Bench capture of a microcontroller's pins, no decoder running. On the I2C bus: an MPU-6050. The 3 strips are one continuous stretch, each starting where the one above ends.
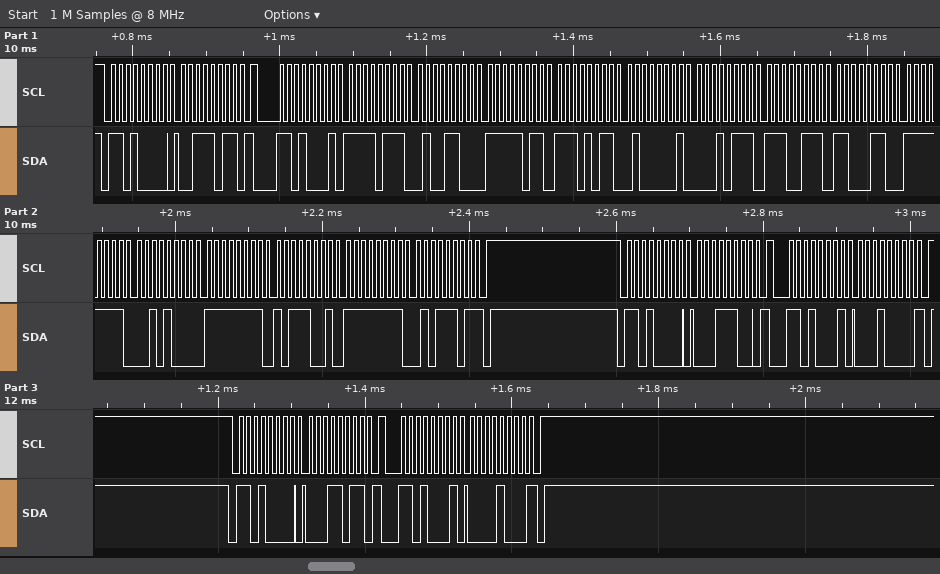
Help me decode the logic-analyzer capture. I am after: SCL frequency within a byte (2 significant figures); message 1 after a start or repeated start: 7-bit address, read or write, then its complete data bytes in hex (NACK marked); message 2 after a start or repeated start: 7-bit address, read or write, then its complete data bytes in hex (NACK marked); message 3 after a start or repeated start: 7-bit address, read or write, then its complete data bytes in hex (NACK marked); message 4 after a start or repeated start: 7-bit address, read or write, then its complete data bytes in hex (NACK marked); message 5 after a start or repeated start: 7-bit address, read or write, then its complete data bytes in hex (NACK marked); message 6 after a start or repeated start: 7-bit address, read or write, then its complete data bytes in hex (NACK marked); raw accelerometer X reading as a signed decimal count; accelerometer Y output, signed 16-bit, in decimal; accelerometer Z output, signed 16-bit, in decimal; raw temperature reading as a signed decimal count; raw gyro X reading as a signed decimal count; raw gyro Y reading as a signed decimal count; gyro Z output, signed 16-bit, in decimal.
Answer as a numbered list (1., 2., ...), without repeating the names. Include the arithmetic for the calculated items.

1. 100 kHz
2. 0x68 write: 3B
3. 0x68 read: F7 4C FB EB 41 17 E7 C6 FF 28 FF B9 FF 5D NACK
4. 0x68 write: 1C
5. 0x68 read: 10 NACK
6. 0x68 write: 1B
7. 0x68 read: 08 NACK
8. 0xF74C = -2228
9. 0xFBEB = -1045
10. 0x4117 = 16663
11. 0xE7C6 = -6202
12. 0xFF28 = -216
13. 0xFFB9 = -71
14. 0xFF5D = -163
